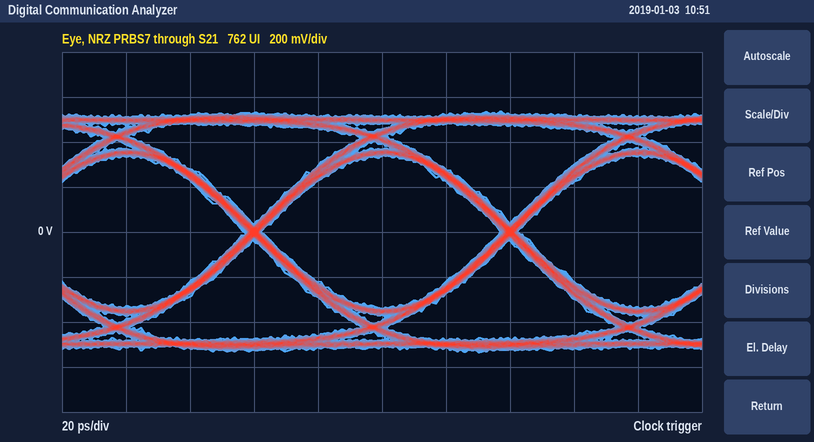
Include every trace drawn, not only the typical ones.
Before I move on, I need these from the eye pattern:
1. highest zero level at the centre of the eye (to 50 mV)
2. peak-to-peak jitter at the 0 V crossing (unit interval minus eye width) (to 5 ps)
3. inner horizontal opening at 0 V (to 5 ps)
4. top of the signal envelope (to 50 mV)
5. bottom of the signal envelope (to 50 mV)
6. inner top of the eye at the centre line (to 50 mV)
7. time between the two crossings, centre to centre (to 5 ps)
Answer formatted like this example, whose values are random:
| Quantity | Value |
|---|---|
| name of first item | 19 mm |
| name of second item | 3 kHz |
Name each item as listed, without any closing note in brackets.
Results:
| Quantity | Value |
|---|---|
| highest zero level at the centre of the eye | -350 mV |
| peak-to-peak jitter at the 0 V crossing (unit interval minus eye width) | 5 ps |
| inner horizontal opening at 0 V | 75 ps |
| top of the signal envelope | 550 mV |
| bottom of the signal envelope | -550 mV |
| inner top of the eye at the centre line | 350 mV |
| time between the two crossings, centre to centre | 80 ps |
